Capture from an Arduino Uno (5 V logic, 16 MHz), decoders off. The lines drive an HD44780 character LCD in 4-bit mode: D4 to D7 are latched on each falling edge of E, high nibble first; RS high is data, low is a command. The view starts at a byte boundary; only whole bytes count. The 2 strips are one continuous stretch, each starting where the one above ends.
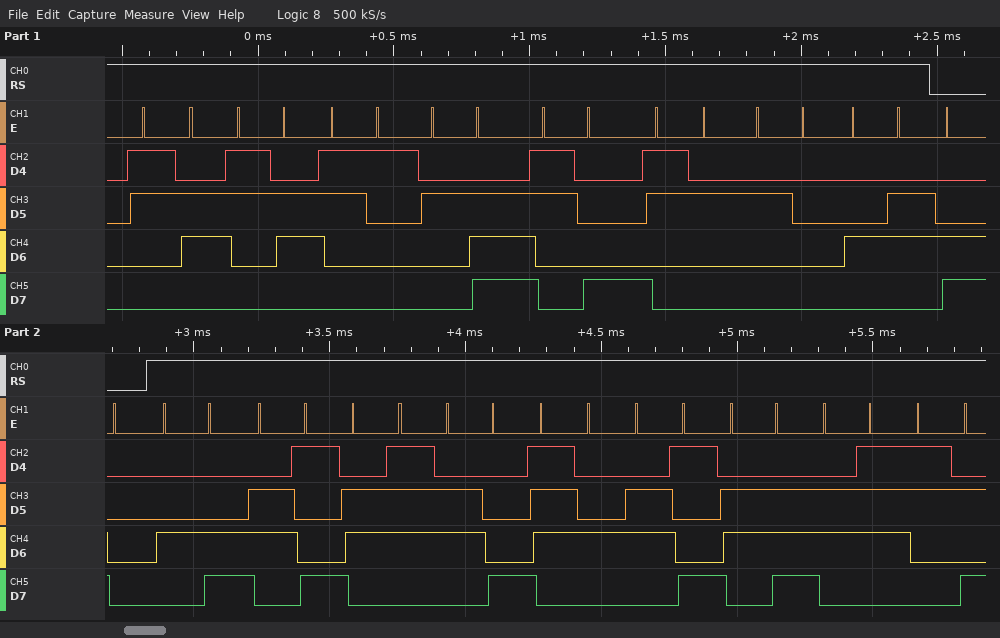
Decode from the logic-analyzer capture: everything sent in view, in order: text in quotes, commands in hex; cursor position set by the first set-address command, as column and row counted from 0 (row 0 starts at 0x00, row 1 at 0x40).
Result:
"661.82 F" 0xC0 "Lighting:"
column 0, row 1
